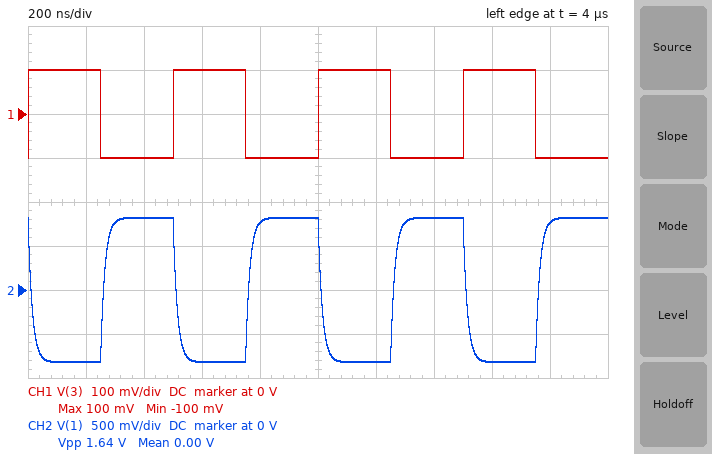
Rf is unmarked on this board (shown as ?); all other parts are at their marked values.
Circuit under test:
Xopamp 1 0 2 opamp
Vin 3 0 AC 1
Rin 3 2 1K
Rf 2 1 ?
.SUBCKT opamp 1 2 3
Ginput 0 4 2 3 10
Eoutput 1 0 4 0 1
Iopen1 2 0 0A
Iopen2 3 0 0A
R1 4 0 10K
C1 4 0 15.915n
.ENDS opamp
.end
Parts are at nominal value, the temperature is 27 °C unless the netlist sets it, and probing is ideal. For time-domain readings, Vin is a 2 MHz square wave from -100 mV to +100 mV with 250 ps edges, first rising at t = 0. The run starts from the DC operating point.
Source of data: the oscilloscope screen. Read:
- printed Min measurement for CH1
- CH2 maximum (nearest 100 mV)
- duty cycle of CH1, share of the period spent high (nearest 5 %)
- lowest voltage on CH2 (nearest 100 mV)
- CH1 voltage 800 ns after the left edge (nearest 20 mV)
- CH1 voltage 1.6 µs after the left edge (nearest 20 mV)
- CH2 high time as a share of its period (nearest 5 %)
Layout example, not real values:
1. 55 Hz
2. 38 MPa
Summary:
1. -100 mV
2. 800 mV
3. 50 %
4. -800 mV
5. -100 mV
6. 100 mV
7. 50 %
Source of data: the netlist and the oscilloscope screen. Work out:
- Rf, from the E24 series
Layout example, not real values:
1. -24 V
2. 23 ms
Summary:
1. 8.2 kΩ
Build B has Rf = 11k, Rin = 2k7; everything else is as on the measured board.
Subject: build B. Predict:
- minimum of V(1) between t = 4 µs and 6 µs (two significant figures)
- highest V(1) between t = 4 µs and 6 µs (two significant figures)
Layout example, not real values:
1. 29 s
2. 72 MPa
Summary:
1. -410 mV
2. 410 mV
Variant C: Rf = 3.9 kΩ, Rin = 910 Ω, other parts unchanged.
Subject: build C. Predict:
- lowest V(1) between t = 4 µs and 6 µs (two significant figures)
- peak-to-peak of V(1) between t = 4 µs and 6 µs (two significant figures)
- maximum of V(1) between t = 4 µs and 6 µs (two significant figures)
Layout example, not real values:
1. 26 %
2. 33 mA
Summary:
1. -430 mV
2. 860 mV
3. 430 mV
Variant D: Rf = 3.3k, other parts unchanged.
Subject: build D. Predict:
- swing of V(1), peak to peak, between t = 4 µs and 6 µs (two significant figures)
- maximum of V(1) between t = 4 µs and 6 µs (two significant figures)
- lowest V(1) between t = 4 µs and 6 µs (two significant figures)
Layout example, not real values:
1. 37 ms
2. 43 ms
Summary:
1. 660 mV
2. 330 mV
3. -330 mV
